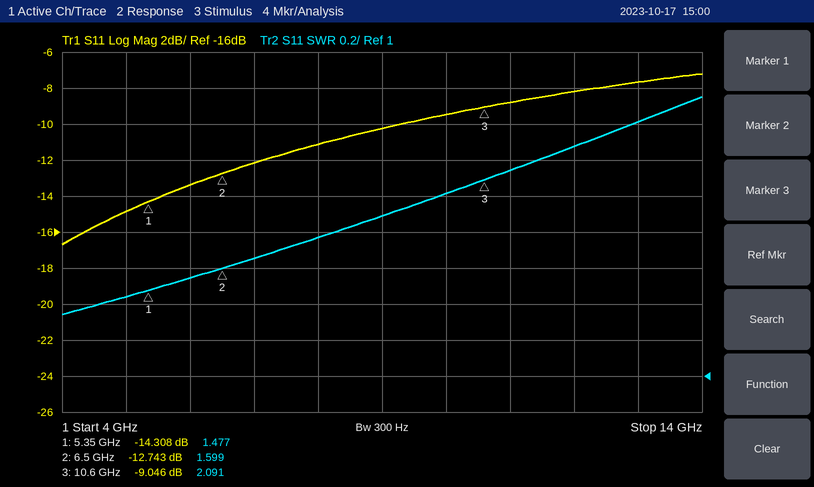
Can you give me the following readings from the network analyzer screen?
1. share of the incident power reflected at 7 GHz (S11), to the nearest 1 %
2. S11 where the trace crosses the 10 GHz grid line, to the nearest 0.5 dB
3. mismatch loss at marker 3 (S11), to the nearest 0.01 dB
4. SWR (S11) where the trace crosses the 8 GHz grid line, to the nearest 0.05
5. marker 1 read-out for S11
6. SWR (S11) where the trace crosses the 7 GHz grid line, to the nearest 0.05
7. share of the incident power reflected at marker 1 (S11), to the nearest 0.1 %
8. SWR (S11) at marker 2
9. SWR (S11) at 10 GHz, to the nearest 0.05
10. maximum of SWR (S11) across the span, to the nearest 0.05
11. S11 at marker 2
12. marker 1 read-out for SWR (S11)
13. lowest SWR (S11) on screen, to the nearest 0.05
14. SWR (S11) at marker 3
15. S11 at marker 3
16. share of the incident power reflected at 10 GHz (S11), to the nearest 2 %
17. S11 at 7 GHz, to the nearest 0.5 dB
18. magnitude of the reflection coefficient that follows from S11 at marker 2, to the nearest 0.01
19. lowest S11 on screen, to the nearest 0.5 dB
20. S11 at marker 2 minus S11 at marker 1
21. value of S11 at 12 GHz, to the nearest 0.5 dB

6 %
-9.5 dB
0.58 dB
1.75
-14.308 dB
1.65
3.7 %
1.599
2.00
2.55
-12.743 dB
1.477
1.35
2.091
-9.046 dB
12 %
-12.0 dB
0.23
-16.5 dB
1.565 dB
-8.0 dB
